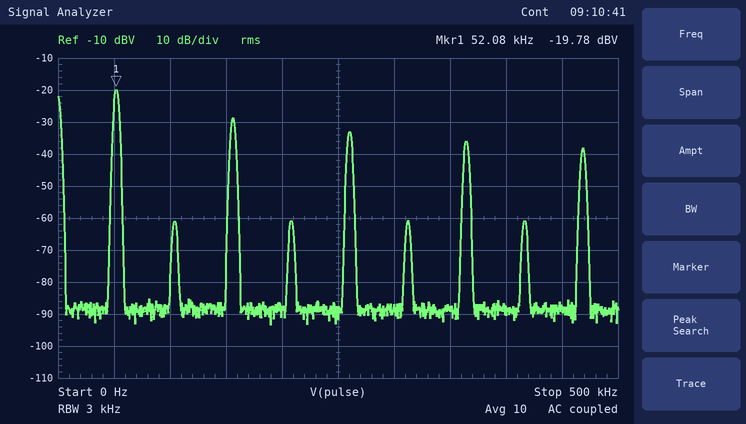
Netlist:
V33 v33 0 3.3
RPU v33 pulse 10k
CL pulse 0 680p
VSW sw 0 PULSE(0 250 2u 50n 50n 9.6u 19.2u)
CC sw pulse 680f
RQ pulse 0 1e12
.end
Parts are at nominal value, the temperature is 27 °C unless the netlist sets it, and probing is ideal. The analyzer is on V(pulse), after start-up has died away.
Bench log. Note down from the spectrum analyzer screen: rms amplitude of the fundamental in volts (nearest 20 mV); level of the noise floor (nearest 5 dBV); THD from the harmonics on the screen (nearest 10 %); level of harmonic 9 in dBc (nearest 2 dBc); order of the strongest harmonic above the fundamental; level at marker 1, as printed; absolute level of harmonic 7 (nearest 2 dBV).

100 mV
-90 dBV
50 %
-18 dBc
3
-19.78 dBV
-36 dBV
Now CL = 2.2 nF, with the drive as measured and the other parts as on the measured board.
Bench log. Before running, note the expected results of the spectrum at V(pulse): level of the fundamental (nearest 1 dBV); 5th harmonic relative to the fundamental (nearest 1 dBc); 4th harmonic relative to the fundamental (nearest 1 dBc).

-29 dBV
-14 dBc
-42 dBc
